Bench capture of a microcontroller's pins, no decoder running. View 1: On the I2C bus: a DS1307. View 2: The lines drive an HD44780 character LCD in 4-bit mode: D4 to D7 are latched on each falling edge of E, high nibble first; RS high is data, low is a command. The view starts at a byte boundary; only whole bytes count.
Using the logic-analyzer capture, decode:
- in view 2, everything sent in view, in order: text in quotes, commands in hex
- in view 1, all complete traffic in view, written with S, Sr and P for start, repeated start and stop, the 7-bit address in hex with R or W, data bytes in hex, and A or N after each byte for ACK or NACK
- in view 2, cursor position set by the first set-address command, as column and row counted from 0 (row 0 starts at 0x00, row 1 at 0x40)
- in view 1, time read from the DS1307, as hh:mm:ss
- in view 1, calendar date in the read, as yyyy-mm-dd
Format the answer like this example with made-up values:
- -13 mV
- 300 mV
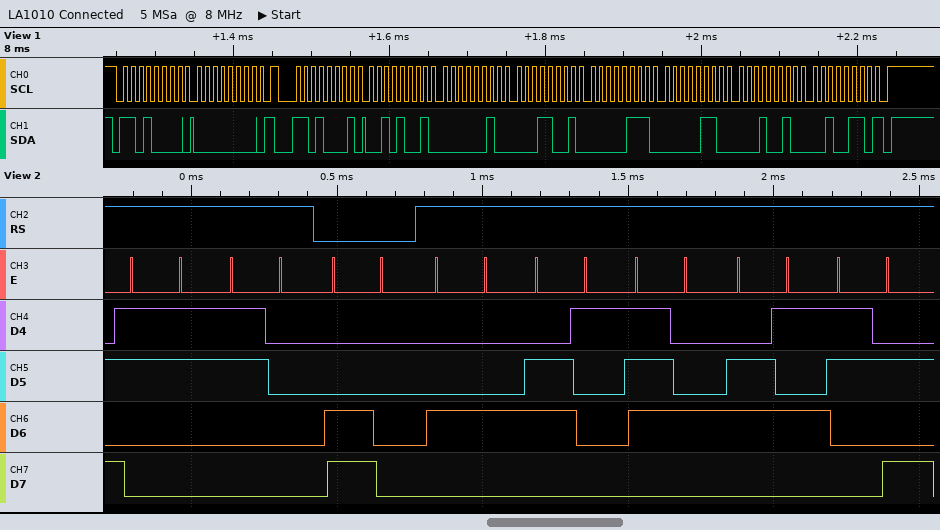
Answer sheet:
- "30" 0xC0 "Date:"
- S 68W A 00 A Sr 68R A 29 A 02 A 19 A 07 A 06 A 12 A 26 N P
- column 0, row 1
- 19:02:29
- 2026-12-06
